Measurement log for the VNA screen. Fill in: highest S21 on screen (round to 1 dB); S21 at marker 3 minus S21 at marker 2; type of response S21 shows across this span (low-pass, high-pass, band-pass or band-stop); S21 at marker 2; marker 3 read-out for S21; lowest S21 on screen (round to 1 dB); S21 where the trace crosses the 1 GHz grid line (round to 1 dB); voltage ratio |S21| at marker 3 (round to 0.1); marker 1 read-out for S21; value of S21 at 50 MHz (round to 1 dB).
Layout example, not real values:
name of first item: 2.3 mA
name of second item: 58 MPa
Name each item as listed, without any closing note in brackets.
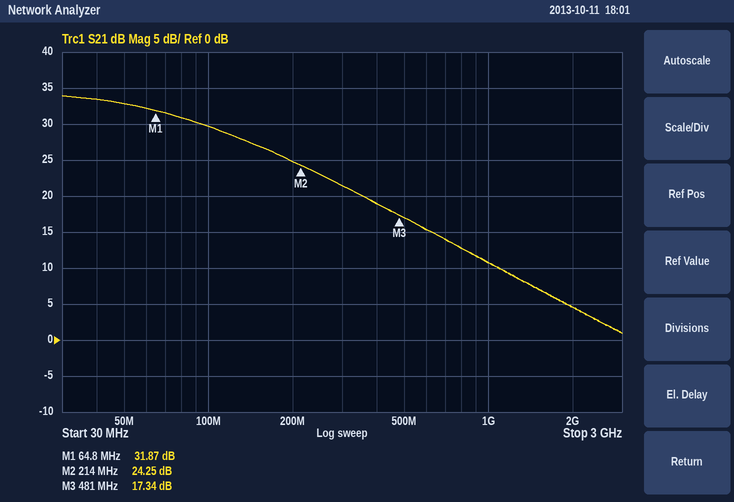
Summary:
highest S21 on screen: 34 dB
S21 at marker 3 minus S21 at marker 2: -6.91 dB
type of response S21 shows across this span: low-pass
S21 at marker 2: 24.25 dB
marker 3 read-out for S21: 17.34 dB
lowest S21 on screen: 1 dB
S21 where the trace crosses the 1 GHz grid line: 11 dB
voltage ratio |S21| at marker 3: 7.4
marker 1 read-out for S21: 31.87 dB
value of S21 at 50 MHz: 33 dB
